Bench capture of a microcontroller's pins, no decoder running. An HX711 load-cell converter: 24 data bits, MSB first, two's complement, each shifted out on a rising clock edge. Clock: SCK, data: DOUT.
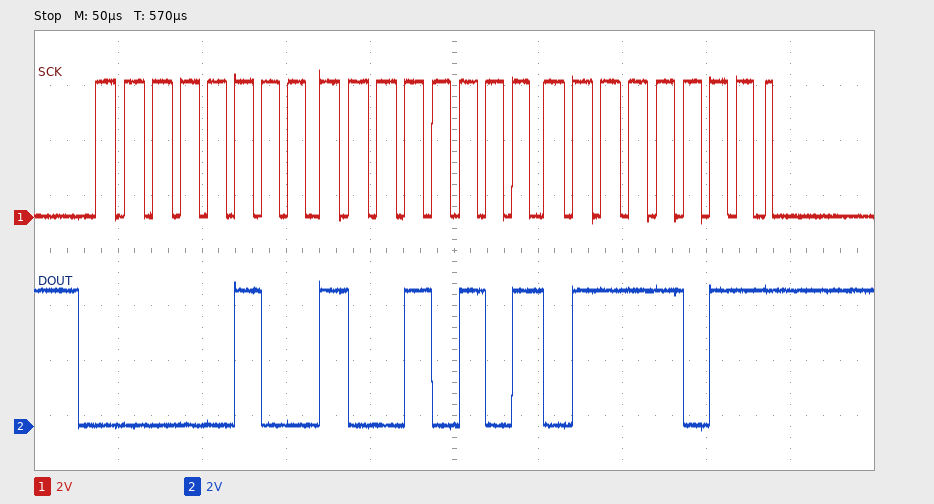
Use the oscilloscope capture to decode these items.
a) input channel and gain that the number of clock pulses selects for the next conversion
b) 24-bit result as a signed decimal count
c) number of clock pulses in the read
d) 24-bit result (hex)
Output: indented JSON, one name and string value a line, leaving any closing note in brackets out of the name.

{
  "input channel and gain that the number of clock pulses selects for the next conversion": "channel A, gain 128",
  "24-bit result as a signed decimal count": "300411",
  "number of clock pulses in the read": "25",
  "24-bit result": "0x04957B"
}
